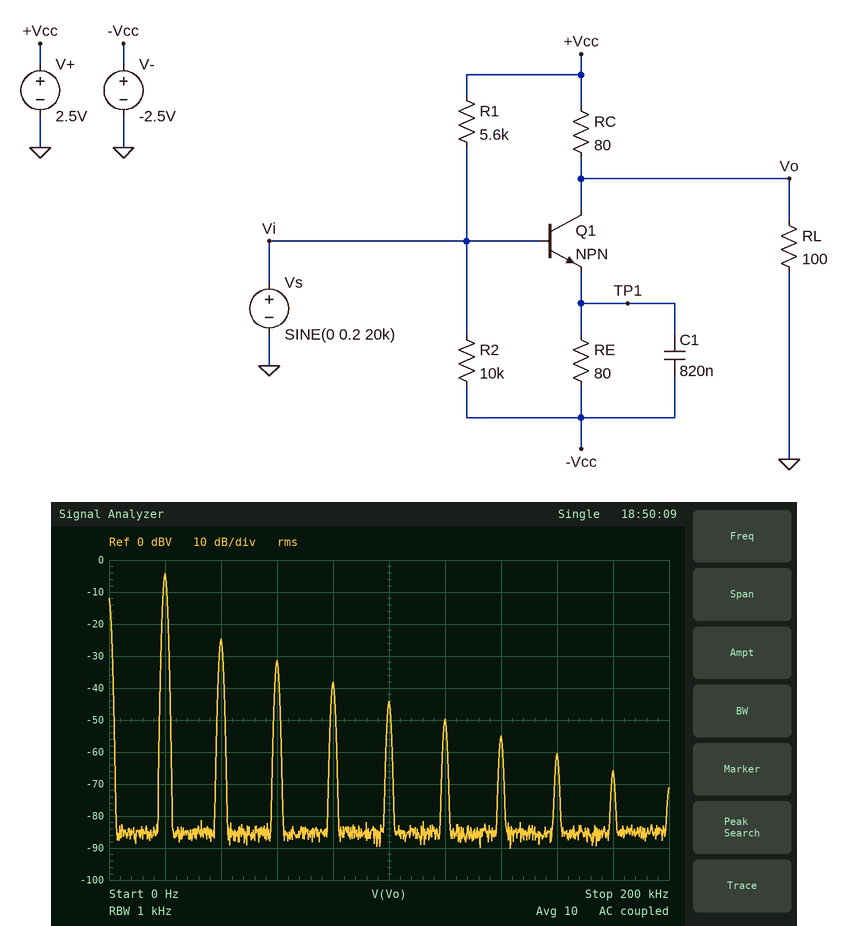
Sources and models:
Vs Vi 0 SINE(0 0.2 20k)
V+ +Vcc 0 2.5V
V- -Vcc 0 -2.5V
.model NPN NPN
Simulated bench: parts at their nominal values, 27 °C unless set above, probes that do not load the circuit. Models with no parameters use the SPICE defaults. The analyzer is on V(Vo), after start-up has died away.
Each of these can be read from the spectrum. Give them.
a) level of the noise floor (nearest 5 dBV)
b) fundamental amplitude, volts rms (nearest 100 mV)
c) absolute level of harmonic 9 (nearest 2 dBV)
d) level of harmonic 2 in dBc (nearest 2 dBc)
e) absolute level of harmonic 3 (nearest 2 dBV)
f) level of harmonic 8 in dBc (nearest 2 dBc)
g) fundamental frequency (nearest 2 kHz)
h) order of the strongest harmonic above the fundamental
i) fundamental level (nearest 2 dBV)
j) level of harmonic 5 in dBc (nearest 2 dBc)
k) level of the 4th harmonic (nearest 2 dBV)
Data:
-85 dBV
600 mV
-66 dBV
-20 dBc
-32 dBV
-56 dBc
20 kHz
2
-4 dBV
-40 dBc
-38 dBV
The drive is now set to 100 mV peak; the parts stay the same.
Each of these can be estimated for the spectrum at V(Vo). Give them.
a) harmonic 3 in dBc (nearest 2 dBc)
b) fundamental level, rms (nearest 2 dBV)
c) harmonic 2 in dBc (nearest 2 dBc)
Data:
-42 dBc
-10 dBV
-30 dBc
